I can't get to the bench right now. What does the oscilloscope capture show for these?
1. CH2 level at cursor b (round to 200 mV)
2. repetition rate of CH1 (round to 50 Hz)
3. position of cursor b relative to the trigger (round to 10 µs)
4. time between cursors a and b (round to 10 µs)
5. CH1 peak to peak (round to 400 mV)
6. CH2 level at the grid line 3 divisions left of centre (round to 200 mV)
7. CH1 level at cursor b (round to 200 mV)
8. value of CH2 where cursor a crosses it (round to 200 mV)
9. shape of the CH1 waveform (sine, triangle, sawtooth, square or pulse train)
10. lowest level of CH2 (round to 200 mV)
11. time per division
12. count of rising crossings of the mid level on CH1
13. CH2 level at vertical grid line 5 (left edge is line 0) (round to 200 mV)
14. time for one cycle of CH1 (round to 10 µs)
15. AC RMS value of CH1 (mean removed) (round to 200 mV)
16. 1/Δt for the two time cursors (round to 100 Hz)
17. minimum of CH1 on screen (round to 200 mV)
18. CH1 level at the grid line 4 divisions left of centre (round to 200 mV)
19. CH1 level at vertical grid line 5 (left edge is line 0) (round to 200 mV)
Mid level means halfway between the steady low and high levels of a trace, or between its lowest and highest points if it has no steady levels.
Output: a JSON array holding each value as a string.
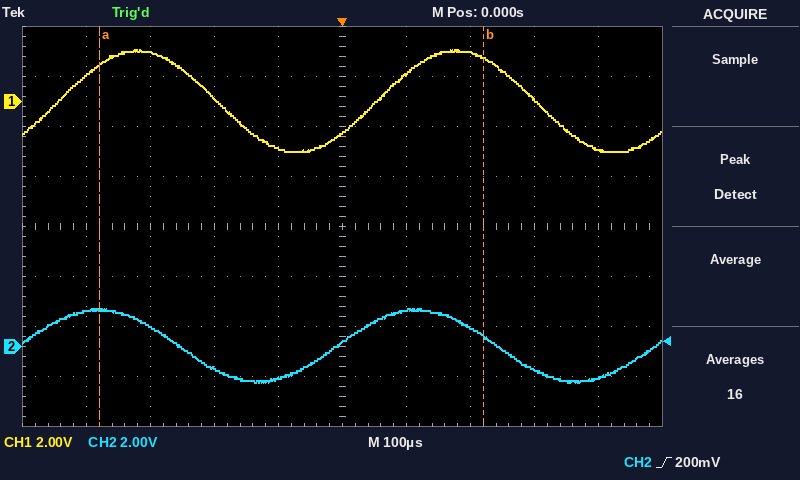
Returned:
["400 mV", "2.00 kHz", "+220 µs", "600 µs", "4.0 V", "800 mV", "1.8 V", "1.4 V", "sine", "-1.4 V", "100 µs", "2", "200 mV", "500 µs", "1.4 V", "1.7 kHz", "-2.0 V", "1.0 V", "-1.2 V"]
